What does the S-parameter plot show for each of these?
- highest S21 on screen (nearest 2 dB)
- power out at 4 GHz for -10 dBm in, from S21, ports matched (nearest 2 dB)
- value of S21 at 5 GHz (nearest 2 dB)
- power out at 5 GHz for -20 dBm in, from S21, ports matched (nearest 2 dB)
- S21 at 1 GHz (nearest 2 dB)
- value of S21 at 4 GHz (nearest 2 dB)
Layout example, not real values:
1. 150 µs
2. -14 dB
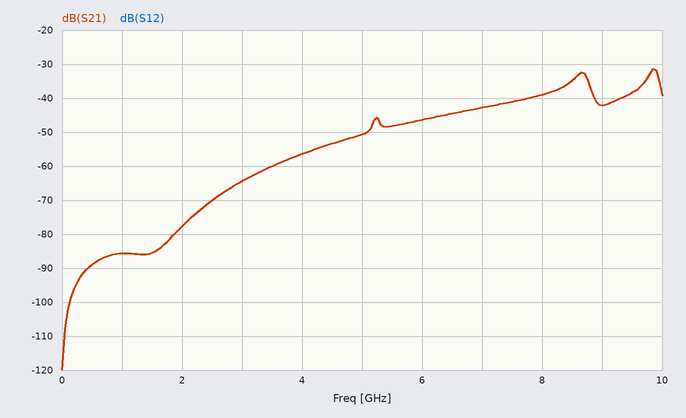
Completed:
1. -32 dB
2. -66 dBm
3. -50 dB
4. -70 dBm
5. -86 dB
6. -56 dB
